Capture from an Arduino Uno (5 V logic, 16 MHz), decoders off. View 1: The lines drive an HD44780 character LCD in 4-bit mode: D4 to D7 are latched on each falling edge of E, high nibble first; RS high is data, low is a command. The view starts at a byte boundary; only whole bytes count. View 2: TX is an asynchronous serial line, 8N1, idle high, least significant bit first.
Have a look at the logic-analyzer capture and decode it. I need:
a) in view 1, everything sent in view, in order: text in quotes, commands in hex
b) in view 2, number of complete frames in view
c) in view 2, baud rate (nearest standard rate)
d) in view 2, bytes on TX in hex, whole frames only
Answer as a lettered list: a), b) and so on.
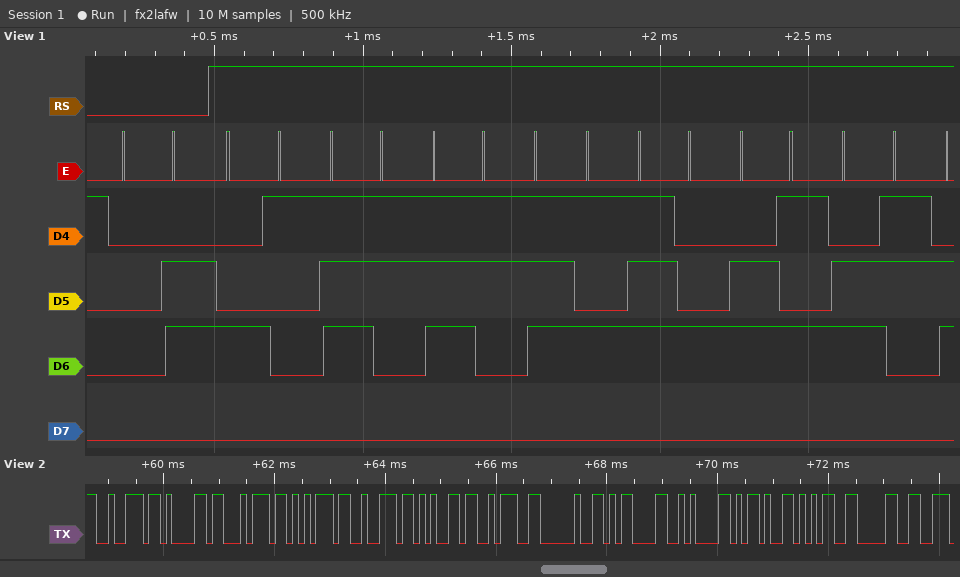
a) 0x06 "Assutec"
b) 13
c) 9600 baud
d) 72 61 74 75 72 65 3A 20 0D 0A 2D 35 30
